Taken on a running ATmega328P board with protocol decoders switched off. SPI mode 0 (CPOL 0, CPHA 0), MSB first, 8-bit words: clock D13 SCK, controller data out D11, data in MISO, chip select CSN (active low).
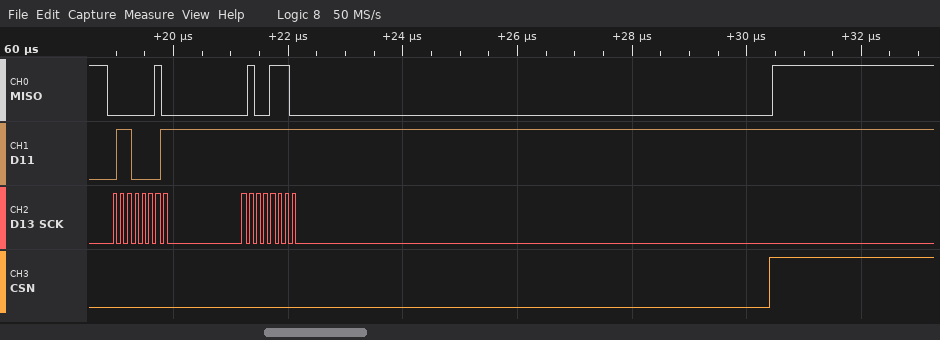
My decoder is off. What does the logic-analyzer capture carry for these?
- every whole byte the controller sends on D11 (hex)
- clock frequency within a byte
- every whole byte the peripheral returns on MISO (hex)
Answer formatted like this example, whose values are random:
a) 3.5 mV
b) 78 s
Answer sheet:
a) 61 FF
b) 8 MHz
c) 02 4E
